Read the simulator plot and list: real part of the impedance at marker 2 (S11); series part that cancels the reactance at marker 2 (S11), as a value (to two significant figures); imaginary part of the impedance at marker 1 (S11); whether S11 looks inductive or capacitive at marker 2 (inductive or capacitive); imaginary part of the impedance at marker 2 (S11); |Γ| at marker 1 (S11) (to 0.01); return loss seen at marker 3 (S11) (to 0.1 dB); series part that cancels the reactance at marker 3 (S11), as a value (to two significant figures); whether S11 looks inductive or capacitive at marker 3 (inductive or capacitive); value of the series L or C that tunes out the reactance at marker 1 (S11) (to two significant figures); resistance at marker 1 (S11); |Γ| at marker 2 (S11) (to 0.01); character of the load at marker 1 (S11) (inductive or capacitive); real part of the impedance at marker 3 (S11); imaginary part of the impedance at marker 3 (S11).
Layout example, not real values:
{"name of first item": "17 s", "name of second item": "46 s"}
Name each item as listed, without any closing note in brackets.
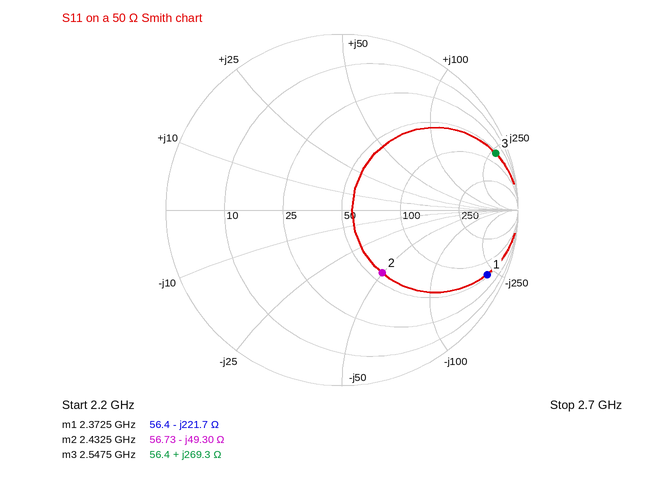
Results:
{"real part of the impedance at marker 2": "56.73 Ω", "series part that cancels the reactance at marker 2 (S11), as a value": "3.2 nH", "imaginary part of the impedance at marker 1": "-221.7 Ω", "whether S11 looks inductive or capacitive at marker 2": "capacitive", "imaginary part of the impedance at marker 2": "-49.30 Ω", "|Γ| at marker 1 (S11)": "0.90", "return loss seen at marker 3 (S11)": "0.6 dB", "series part that cancels the reactance at marker 3 (S11), as a value": "230 fF", "whether S11 looks inductive or capacitive at marker 3": "inductive", "value of the series L or C that tunes out the reactance at marker 1 (S11)": "15 nH", "resistance at marker 1": "56.4 Ω", "|Γ| at marker 2 (S11)": "0.42", "character of the load at marker 1 (S11)": "capacitive", "real part of the impedance at marker 3": "56.4 Ω", "imaginary part of the impedance at marker 3": "+269.3 Ω"}
